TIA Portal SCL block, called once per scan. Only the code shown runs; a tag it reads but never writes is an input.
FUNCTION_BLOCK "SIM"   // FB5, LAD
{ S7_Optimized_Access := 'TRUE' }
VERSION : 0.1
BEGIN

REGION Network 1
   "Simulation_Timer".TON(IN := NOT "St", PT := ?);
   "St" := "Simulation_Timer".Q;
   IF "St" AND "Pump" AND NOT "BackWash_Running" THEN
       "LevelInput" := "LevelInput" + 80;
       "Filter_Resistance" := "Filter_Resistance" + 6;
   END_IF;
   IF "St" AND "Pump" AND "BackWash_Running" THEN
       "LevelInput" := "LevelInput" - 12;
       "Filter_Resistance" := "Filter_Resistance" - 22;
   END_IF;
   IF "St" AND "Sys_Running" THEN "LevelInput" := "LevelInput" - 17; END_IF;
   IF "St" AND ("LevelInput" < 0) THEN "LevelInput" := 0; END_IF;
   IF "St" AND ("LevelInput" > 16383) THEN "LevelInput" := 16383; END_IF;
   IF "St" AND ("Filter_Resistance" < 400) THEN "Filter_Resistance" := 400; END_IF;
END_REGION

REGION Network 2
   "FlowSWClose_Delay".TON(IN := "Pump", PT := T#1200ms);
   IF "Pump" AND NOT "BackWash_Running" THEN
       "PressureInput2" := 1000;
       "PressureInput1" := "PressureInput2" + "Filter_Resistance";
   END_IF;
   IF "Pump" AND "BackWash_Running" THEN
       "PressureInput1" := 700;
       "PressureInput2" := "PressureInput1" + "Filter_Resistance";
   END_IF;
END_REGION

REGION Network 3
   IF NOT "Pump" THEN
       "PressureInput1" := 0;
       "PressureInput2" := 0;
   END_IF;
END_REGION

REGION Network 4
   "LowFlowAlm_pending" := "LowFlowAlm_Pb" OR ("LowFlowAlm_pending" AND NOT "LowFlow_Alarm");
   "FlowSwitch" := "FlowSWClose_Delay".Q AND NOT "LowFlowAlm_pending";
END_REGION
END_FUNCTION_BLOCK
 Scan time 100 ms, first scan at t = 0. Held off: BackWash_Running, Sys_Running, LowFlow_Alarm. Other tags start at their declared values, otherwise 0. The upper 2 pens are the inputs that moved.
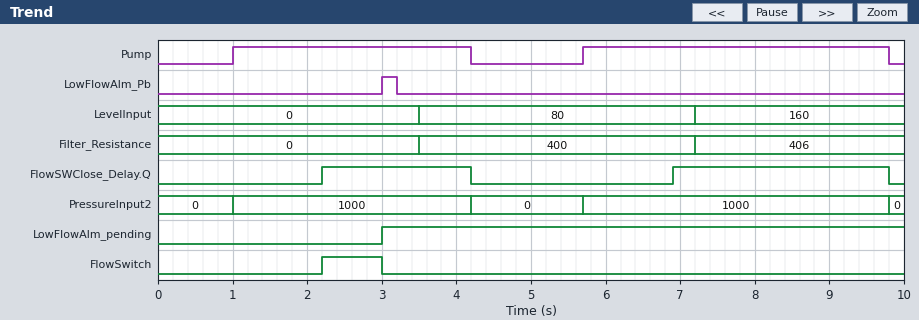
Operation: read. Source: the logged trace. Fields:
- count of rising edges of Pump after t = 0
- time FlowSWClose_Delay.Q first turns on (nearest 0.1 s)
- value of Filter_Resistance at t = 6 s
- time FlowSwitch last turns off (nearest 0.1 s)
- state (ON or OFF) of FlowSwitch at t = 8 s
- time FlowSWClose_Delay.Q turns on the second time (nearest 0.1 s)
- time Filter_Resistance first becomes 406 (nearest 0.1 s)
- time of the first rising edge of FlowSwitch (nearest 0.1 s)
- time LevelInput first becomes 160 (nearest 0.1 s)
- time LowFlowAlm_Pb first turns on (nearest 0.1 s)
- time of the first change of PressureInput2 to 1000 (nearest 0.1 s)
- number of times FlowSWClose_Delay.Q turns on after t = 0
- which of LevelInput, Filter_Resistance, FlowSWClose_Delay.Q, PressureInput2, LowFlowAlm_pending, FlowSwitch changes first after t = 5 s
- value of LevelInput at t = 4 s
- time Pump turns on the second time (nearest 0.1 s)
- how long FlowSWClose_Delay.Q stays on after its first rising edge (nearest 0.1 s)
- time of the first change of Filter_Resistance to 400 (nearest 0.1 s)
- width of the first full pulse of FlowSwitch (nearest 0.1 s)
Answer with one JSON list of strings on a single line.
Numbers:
["2", "2.2 s", "400", "3.0 s", "OFF", "6.9 s", "7.2 s", "2.2 s", "7.2 s", "3.0 s", "1.0 s", "2", "PressureInput2", "80", "5.7 s", "2.0 s", "3.5 s", "0.8 s"]
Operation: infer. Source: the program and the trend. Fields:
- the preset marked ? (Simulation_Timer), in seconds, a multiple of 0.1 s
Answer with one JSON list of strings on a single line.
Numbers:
["3.5 s"]
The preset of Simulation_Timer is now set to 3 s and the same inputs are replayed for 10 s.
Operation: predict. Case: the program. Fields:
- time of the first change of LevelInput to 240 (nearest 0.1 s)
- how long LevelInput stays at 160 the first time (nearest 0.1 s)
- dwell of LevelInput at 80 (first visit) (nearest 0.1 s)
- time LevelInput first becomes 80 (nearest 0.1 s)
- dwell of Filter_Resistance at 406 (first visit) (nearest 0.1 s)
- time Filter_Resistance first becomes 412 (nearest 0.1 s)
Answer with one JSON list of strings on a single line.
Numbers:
["9.4 s", "3.2 s", "3.2 s", "3.0 s", "3.2 s", "9.4 s"]
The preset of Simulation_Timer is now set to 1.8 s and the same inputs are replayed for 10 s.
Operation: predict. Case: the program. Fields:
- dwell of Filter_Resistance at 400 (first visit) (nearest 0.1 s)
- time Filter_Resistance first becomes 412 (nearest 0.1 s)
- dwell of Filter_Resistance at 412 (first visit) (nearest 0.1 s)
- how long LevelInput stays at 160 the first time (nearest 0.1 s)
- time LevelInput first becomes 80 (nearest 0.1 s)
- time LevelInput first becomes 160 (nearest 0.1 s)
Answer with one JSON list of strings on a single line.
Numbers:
["2.0 s", "5.8 s", "2.0 s", "2.0 s", "1.8 s", "3.8 s"]
